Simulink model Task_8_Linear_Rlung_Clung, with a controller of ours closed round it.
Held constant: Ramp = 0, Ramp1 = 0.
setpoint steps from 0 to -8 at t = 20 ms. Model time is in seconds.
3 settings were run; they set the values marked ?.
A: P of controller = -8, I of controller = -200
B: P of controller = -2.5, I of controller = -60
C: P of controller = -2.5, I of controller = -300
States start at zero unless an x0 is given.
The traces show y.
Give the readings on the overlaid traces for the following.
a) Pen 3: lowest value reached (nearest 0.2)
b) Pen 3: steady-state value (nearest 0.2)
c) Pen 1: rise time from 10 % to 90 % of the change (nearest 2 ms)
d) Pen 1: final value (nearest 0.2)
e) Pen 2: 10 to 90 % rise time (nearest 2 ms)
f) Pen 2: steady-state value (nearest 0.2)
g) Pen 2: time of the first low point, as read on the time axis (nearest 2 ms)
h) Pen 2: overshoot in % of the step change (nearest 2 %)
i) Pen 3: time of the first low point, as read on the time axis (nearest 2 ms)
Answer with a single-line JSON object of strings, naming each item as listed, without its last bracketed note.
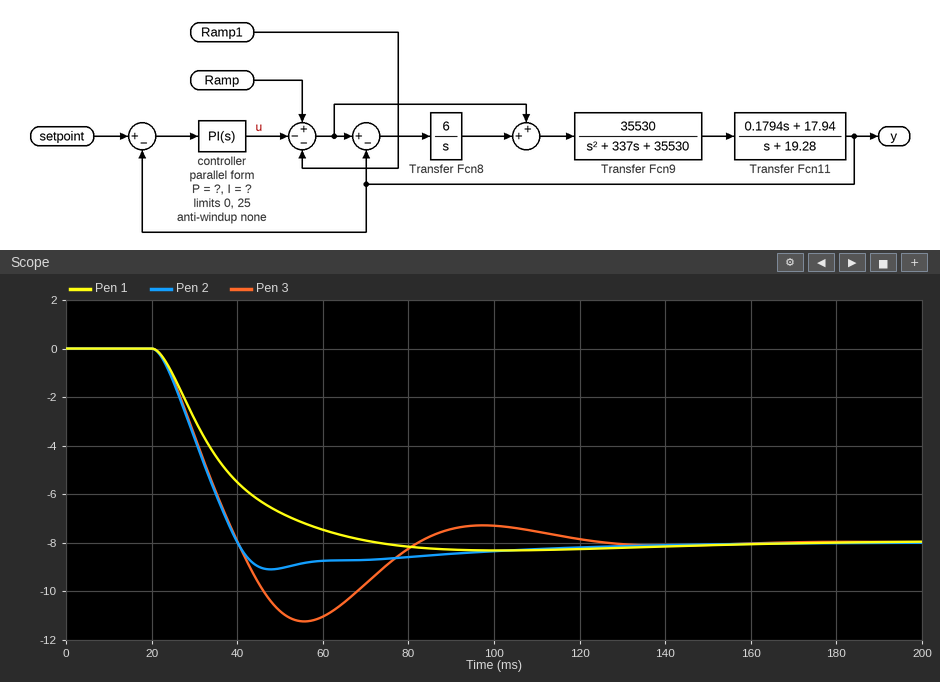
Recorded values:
{"Pen 3: lowest value reached": "-11.2", "Pen 3: steady-state value": "-8.0", "Pen 1: rise time from 10 % to 90 % of the change": "32 ms", "Pen 1: final value": "-8.0", "Pen 2: 10 to 90 % rise time": "14 ms", "Pen 2: steady-state value": "-8.0", "Pen 2: time of the first low point, as read on the time axis": "48 ms", "Pen 2: overshoot in % of the step change": "14 %", "Pen 3: time of the first low point, as read on the time axis": "56 ms"}
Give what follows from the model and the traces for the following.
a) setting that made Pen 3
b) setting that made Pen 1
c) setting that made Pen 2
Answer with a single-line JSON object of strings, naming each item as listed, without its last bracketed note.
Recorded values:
{"setting that made Pen 3": "C", "setting that made Pen 1": "B", "setting that made Pen 2": "A"}
